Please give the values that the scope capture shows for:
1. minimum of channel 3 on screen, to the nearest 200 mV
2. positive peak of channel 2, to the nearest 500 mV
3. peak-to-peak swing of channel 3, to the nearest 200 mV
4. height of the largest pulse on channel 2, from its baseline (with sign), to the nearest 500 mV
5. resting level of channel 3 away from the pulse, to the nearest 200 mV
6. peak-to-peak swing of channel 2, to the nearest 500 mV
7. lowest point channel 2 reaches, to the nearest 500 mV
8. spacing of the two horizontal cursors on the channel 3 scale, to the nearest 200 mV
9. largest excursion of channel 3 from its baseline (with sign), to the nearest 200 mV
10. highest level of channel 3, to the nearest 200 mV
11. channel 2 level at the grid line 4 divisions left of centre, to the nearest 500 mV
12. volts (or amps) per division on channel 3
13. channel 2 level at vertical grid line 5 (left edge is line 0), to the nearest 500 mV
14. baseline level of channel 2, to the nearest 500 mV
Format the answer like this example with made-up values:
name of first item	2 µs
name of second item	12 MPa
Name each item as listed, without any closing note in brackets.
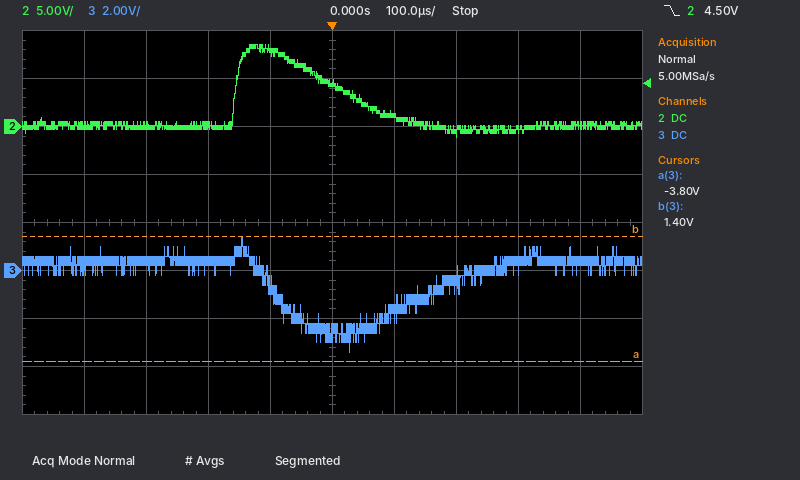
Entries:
minimum of channel 3 on screen, to the nearest 200 mV	-3.4 V
positive peak of channel 2, to the nearest 500 mV	8.5 V
peak-to-peak swing of channel 3, to the nearest 200 mV	4.8 V
height of the largest pulse on channel 2, from its baseline (with sign), to the nearest 500 mV	+8.5 V
resting level of channel 3 away from the pulse, to the nearest 200 mV	400 mV
peak-to-peak swing of channel 2, to the nearest 500 mV	9.5 V
lowest point channel 2 reaches, to the nearest 500 mV	-1.0 V
spacing of the two horizontal cursors on the channel 3 scale, to the nearest 200 mV	5.2 V
largest excursion of channel 3 from its baseline (with sign), to the nearest 200 mV	-3.8 V
highest level of channel 3, to the nearest 200 mV	1.4 V
channel 2 level at the grid line 4 divisions left of centre, to the nearest 500 mV	0.0 V
volts (or amps) per division on channel 3	2 V
channel 2 level at vertical grid line 5 (left edge is line 0), to the nearest 500 mV	4.5 V
baseline level of channel 2, to the nearest 500 mV	0.0 V
